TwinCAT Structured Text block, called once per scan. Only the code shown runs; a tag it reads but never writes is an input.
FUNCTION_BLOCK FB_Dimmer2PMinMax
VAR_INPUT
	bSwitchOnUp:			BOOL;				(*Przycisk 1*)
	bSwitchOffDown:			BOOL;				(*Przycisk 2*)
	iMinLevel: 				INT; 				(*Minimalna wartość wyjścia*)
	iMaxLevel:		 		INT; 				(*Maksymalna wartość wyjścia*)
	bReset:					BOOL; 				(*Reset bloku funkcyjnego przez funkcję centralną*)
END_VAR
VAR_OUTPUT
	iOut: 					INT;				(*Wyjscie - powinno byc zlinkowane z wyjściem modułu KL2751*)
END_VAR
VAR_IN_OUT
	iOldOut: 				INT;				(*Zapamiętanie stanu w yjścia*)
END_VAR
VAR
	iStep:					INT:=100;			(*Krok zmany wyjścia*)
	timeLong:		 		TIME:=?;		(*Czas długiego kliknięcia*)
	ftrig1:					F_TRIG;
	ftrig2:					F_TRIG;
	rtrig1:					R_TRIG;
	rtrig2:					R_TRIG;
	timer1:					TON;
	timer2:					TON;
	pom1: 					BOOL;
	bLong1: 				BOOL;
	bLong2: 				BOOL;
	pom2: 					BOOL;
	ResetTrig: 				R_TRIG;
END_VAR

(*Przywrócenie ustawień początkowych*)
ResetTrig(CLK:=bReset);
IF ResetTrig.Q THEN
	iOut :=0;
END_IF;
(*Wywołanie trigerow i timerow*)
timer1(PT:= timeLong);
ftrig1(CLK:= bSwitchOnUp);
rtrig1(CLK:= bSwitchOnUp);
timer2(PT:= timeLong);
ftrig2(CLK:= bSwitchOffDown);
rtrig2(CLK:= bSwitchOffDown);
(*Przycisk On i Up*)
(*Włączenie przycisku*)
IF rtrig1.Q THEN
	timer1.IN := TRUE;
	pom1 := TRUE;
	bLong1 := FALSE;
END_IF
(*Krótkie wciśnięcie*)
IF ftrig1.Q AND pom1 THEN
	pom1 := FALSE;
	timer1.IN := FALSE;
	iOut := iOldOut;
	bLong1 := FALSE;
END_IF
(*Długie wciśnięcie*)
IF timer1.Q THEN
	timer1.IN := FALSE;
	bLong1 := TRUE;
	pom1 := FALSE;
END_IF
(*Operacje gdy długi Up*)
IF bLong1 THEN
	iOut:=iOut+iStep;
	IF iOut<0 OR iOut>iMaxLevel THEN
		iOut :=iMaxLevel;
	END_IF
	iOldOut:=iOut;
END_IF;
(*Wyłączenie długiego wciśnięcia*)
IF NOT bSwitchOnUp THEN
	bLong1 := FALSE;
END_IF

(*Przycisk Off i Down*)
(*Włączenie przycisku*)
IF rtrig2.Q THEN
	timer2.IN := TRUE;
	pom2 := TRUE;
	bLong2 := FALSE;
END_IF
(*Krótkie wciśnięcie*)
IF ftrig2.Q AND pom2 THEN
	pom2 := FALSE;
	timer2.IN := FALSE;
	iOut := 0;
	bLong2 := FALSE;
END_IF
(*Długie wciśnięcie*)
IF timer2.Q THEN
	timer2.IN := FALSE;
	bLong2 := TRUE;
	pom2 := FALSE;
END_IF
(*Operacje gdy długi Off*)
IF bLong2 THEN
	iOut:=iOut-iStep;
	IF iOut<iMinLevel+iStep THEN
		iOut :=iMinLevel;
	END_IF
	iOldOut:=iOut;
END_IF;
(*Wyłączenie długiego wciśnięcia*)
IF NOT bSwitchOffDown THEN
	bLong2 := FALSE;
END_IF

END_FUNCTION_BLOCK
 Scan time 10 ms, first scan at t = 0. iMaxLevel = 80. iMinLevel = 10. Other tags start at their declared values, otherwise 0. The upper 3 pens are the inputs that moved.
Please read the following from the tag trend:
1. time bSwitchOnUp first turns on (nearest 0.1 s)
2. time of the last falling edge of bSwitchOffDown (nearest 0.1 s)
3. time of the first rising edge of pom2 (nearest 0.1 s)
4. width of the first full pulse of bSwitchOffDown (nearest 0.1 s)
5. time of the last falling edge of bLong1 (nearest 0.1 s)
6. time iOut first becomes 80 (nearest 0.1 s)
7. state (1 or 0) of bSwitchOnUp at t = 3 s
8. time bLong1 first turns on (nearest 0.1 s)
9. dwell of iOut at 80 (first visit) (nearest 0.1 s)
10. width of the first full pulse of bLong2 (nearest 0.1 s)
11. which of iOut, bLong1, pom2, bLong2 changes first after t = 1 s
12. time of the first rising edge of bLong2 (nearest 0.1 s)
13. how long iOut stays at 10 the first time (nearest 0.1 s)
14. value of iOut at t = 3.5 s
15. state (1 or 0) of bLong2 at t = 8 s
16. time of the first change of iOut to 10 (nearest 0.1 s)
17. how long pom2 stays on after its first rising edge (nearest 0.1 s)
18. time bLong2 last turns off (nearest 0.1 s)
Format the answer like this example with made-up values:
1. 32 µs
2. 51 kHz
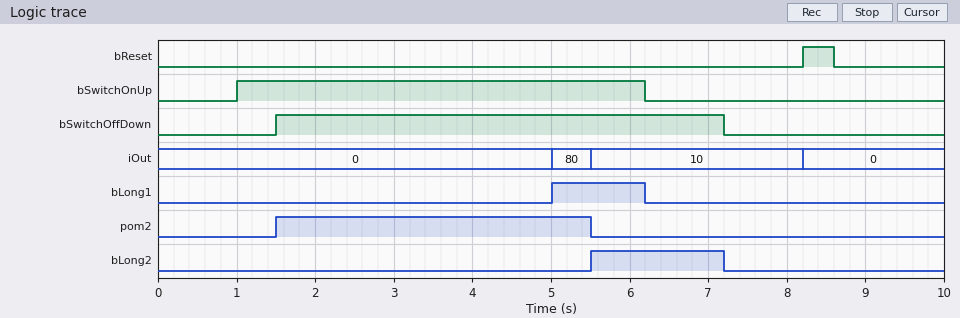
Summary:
1. 1.0 s
2. 7.2 s
3. 1.5 s
4. 5.7 s
5. 6.2 s
6. 5.0 s
7. 1
8. 5.0 s
9. 0.5 s
10. 1.7 s
11. pom2
12. 5.5 s
13. 2.7 s
14. 0
15. 0
16. 5.5 s
17. 4.0 s
18. 7.2 s
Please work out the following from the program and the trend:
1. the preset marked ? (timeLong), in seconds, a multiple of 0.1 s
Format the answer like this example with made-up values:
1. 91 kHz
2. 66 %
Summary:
1. 4.0 s
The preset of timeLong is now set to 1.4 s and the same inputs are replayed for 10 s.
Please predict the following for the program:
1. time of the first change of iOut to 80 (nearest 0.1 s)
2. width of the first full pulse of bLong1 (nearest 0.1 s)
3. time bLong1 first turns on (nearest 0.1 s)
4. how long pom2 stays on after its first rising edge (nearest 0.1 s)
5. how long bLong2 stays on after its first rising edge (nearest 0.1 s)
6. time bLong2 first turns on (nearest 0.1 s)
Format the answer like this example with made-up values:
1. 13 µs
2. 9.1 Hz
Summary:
1. 2.4 s
2. 3.8 s
3. 2.4 s
4. 1.4 s
5. 4.3 s
6. 2.9 s
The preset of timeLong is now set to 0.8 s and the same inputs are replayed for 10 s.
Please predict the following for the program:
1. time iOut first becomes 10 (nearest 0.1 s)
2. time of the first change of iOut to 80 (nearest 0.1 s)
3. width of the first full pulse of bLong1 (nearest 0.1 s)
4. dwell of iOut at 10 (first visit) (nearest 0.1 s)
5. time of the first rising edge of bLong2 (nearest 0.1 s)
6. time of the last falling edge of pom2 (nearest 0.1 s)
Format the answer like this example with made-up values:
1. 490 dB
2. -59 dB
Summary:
1. 2.3 s
2. 1.8 s
3. 4.4 s
4. 5.9 s
5. 2.3 s
6. 2.3 s
